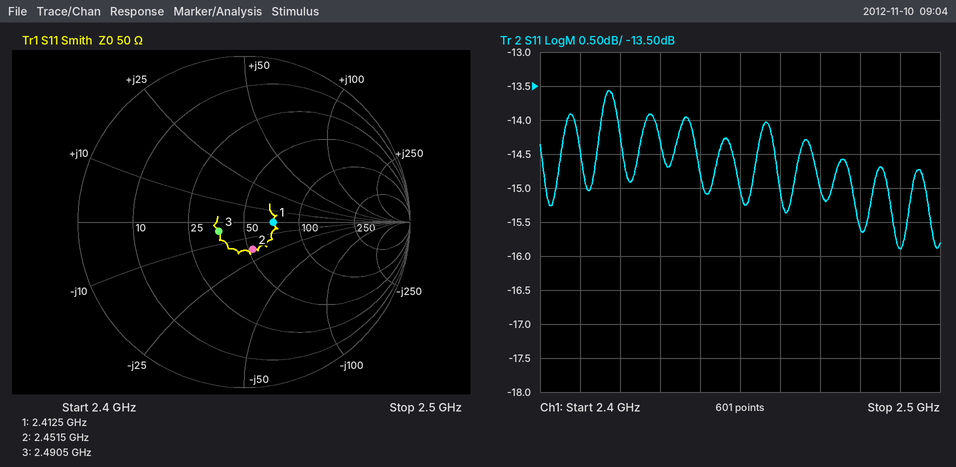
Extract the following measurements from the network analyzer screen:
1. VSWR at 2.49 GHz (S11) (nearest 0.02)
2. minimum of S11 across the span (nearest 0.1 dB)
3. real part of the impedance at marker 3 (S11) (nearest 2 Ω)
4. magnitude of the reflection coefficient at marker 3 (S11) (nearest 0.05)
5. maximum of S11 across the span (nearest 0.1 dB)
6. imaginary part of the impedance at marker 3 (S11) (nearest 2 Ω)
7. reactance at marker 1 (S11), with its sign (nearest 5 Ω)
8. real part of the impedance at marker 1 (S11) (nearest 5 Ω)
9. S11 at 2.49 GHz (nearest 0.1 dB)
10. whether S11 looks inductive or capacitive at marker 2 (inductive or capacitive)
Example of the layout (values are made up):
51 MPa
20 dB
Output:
1.38
-15.9 dB
36 Ω
0.15
-13.6 dB
-4 Ω
0 Ω
70 Ω
-15.9 dB
capacitive
